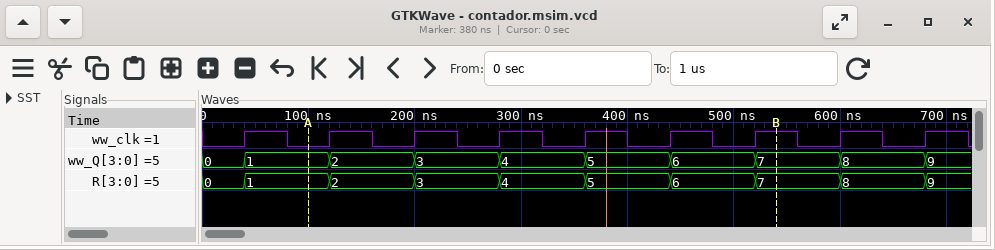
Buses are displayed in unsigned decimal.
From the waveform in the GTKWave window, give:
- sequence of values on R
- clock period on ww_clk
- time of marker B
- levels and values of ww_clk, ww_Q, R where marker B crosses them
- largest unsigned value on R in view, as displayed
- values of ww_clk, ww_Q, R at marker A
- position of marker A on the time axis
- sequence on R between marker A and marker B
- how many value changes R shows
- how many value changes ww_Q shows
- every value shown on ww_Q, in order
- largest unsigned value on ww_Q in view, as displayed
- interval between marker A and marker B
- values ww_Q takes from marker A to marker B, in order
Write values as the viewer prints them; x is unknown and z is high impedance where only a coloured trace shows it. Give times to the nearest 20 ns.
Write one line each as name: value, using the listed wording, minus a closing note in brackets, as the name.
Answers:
sequence of values on R: 0, 1, 2, 3, 4, 5, 6, 7, 8, 9
clock period on ww_clk: 80 ns
time of marker B: 540 ns
levels and values of ww_clk, ww_Q, R where marker B crosses them: ww_clk=1, ww_Q=7, R=7
largest unsigned value on R in view, as displayed: 9
values of ww_clk, ww_Q, R at marker A: ww_clk=0, ww_Q=1, R=1
position of marker A on the time axis: 100 ns
sequence on R between marker A and marker B: 1, 2, 3, 4, 5, 6, 7
how many value changes R shows: 9
how many value changes ww_Q shows: 9
every value shown on ww_Q, in order: 0, 1, 2, 3, 4, 5, 6, 7, 8, 9
largest unsigned value on ww_Q in view, as displayed: 9
interval between marker A and marker B: 440 ns
values ww_Q takes from marker A to marker B, in order: 1, 2, 3, 4, 5, 6, 7
